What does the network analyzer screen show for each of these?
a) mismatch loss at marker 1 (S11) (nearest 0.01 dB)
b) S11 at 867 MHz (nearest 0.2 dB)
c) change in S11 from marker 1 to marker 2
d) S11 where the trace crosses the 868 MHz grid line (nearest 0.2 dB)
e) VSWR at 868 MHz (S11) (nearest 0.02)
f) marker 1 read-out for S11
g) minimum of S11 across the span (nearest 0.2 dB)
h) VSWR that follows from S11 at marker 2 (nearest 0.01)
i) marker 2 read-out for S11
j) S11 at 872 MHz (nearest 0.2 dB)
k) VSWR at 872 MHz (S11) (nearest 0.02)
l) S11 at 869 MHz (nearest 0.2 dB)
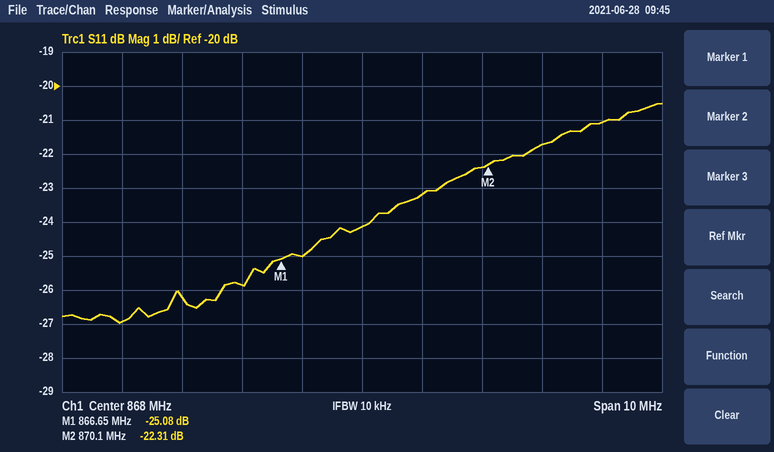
0.01 dB
-25.0 dB
2.77 dB
-24.2 dB
1.14
-25.08 dB
-27.0 dB
1.17
-22.31 dB
-21.0 dB
1.20
-23.2 dB
